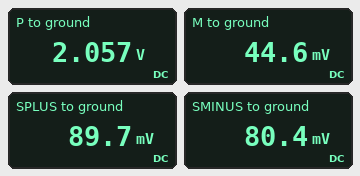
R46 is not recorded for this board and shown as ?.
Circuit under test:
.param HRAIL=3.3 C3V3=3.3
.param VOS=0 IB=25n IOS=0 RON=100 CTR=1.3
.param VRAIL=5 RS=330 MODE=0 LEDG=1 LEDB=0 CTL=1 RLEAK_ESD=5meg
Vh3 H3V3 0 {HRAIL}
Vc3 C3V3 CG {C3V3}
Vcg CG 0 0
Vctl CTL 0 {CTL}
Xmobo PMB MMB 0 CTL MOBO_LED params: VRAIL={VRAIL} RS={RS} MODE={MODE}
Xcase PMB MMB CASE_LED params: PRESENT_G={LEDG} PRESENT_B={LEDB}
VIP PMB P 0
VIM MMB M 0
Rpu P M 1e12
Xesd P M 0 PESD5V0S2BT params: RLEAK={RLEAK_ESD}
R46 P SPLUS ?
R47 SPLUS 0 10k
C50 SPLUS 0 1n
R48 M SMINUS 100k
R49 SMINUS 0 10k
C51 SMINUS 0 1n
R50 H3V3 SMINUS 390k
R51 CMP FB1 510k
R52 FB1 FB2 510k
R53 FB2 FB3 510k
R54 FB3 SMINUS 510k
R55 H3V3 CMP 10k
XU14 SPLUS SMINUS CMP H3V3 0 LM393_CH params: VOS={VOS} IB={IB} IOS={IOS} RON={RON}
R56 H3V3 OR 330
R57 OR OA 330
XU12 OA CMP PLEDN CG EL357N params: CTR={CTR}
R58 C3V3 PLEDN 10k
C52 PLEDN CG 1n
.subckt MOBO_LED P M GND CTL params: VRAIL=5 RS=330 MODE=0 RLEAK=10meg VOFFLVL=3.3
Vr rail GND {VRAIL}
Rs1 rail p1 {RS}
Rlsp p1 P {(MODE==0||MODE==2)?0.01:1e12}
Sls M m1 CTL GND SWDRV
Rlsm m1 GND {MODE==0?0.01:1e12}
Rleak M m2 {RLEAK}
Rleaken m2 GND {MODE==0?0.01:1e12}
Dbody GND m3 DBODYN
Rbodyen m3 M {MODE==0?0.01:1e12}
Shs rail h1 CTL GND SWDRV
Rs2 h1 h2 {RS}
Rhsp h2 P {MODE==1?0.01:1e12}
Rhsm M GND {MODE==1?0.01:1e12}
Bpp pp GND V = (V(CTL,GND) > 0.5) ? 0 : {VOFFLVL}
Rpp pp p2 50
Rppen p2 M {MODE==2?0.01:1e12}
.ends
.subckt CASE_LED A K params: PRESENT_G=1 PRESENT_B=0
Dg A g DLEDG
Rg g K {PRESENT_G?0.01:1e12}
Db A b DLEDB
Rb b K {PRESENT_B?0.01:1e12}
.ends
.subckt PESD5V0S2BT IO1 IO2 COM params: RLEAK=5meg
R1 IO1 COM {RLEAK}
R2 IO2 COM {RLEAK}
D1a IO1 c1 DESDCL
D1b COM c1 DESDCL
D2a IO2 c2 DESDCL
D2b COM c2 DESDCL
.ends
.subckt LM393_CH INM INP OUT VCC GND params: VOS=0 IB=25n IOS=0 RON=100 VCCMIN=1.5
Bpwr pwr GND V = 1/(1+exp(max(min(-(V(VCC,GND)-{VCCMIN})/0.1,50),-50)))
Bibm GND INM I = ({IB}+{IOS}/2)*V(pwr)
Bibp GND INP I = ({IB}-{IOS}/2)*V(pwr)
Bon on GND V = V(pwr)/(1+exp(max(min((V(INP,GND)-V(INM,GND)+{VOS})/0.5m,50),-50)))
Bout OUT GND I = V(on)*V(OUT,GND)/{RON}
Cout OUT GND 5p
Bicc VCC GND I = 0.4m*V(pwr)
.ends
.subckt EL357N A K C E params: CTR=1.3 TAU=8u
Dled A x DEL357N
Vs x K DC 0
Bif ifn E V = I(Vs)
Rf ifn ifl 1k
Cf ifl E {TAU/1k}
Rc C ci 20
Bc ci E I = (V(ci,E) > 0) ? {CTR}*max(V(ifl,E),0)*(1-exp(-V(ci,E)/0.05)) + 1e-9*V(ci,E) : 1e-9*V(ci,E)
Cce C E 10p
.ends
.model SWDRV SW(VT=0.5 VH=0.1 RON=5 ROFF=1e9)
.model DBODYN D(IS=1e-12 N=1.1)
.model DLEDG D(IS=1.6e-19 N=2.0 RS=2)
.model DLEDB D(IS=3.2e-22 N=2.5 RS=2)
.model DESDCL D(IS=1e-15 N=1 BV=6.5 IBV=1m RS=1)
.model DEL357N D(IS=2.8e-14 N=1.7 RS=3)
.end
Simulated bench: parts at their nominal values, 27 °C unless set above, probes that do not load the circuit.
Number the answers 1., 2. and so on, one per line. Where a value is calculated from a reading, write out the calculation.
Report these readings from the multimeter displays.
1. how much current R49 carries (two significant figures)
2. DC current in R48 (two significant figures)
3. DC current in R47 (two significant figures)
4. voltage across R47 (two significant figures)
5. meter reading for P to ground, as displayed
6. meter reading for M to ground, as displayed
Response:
1. (80.4 mV) / 10 kΩ = 8.0 µA
2. (80.4 mV - 44.6 mV) / 100 kΩ = 360 nA
3. (89.7 mV) / 10 kΩ = 9.0 µA
4. 89.7 mV = 90 mV
5. 2.057 V
6. 44.6 mV
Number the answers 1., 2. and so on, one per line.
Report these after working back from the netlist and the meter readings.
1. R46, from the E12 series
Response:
1. 220 kΩ
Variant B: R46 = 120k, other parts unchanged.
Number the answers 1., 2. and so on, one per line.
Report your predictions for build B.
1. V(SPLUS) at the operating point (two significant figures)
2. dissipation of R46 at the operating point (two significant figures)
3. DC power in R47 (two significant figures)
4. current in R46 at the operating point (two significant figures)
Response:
1. 160 mV
2. 30 µW
3. 2.5 µW
4. 16 µA
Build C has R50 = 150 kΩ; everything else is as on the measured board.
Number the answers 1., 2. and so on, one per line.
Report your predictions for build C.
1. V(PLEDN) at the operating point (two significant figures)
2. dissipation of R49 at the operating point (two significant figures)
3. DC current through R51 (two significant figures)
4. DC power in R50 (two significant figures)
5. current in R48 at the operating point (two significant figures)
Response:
1. 3.3 V
2. 4.2 µW
3. 1.5 µA
4. 64 µW
5. 1.6 µA
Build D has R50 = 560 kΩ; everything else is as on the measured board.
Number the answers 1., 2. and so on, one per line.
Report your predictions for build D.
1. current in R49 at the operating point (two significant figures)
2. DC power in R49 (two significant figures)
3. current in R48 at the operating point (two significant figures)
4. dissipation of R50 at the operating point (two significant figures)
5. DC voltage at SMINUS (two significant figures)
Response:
1. 5.8 µA
2. 340 nW
3. 130 nA
4. 19 µW
5. 58 mV
